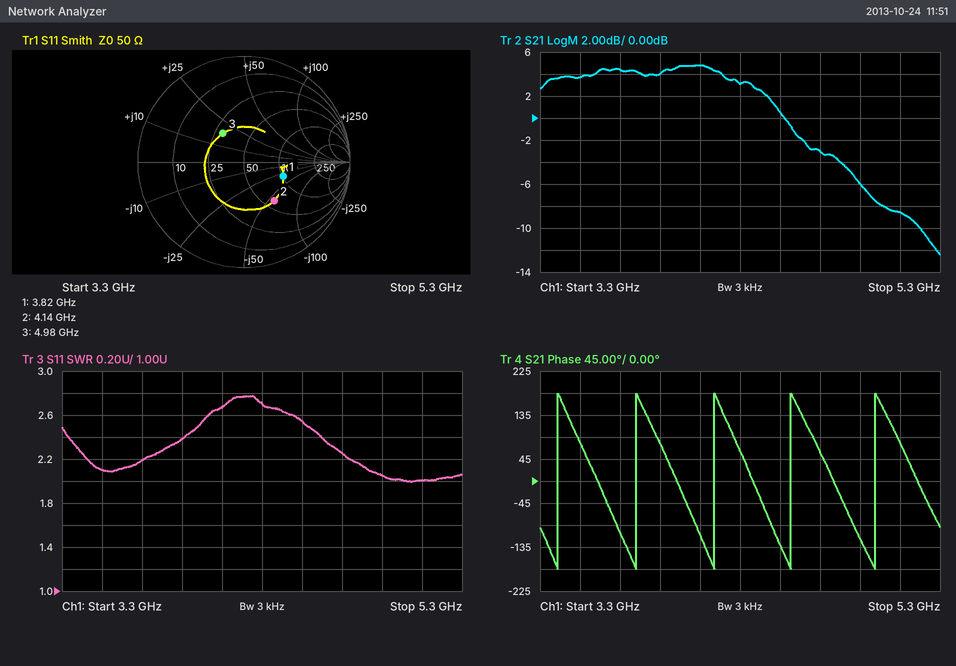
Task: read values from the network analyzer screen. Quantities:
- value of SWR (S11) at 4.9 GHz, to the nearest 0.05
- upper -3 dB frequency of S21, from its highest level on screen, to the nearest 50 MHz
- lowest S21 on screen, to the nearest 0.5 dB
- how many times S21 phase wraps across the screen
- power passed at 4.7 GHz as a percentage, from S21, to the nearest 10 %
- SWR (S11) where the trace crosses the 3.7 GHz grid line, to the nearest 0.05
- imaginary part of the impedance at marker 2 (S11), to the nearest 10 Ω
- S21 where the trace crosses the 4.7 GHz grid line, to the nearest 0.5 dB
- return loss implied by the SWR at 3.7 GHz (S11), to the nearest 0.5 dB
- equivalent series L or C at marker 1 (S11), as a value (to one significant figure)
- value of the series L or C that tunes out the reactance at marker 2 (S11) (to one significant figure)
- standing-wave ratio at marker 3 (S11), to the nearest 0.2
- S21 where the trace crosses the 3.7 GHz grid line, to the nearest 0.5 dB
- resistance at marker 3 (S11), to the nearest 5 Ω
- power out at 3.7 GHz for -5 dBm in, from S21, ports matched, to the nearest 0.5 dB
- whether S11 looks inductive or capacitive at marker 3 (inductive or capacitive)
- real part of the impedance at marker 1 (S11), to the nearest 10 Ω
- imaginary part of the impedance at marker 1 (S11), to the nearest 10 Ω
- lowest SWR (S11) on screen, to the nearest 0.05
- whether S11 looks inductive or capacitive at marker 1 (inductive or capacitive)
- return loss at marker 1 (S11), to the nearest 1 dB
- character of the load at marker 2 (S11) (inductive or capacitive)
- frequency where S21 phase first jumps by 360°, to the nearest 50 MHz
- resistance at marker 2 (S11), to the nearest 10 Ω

2.05
4.45 GHz
-12.5 dB
5
50 %
2.20
-60 Ω
-3.0 dB
8.5 dB
1 pF
2 nH
2.0
4.5 dB
30 Ω
-0.5 dBm
inductive
100 Ω
-30 Ω
2.00
capacitive
8 dB
capacitive
3.40 GHz
60 Ω
